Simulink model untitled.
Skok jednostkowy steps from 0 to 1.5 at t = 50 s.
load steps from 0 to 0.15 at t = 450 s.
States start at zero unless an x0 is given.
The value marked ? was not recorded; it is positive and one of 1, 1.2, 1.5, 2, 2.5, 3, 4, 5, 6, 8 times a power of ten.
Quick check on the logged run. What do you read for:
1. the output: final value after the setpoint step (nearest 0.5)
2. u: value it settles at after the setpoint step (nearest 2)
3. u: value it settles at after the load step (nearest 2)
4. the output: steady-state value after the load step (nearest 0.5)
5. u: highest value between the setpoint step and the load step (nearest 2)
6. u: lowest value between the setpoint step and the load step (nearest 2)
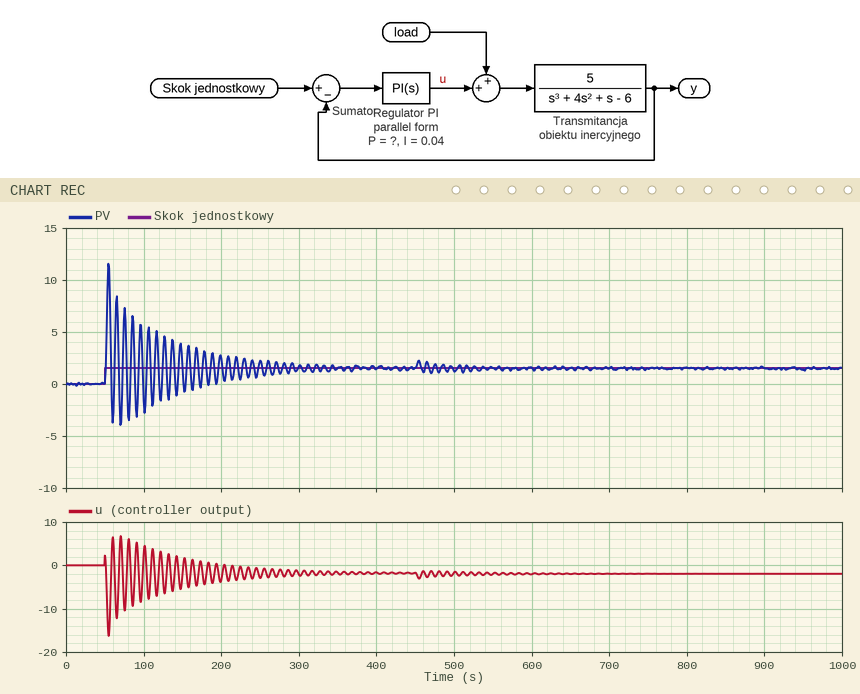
1.5
-2
-2
1.5
6
-16
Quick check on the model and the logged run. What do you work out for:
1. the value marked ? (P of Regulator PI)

1.5
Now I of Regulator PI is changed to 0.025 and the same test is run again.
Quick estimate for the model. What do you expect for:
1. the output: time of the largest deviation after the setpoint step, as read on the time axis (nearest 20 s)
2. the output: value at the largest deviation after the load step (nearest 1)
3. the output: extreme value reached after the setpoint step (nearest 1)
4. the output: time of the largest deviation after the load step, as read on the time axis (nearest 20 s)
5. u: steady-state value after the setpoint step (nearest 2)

60 s
2
12
460 s
-2
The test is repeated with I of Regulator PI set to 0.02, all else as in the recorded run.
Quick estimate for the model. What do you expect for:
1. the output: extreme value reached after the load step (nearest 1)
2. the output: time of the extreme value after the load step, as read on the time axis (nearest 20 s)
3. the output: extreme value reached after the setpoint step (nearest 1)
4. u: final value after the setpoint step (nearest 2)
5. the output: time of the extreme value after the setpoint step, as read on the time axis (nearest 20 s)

2
460 s
12
-2
60 s
